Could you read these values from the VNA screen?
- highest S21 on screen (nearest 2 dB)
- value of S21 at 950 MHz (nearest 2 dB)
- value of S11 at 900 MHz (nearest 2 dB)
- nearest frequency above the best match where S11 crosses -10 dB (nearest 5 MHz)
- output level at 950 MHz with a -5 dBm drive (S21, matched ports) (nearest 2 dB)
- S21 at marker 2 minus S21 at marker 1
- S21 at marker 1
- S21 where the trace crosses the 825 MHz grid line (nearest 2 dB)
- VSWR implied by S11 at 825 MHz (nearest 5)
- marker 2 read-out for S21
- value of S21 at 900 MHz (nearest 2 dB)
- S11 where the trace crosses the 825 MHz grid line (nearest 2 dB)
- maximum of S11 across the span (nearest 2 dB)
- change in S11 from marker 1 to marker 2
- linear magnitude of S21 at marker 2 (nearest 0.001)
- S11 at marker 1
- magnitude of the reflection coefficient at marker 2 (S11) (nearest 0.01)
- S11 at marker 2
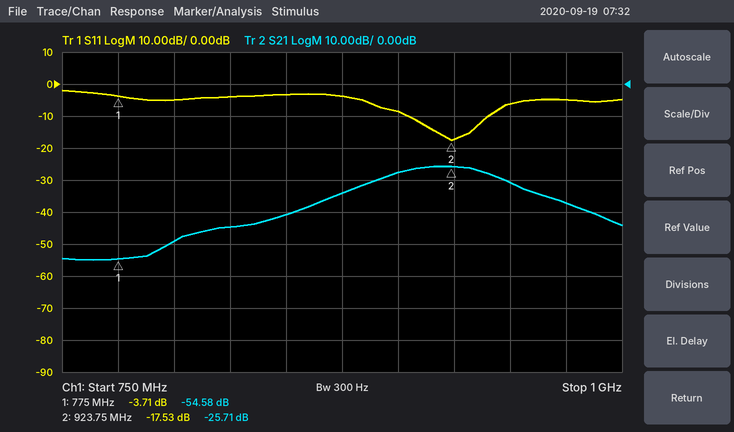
-26 dB
-30 dB
-8 dB
940 MHz
-36 dBm
28.87 dB
-54.58 dB
-44 dB
5
-25.71 dB
-28 dB
-4 dB
-2 dB
-13.82 dB
0.052
-3.71 dB
0.13
-17.53 dB
